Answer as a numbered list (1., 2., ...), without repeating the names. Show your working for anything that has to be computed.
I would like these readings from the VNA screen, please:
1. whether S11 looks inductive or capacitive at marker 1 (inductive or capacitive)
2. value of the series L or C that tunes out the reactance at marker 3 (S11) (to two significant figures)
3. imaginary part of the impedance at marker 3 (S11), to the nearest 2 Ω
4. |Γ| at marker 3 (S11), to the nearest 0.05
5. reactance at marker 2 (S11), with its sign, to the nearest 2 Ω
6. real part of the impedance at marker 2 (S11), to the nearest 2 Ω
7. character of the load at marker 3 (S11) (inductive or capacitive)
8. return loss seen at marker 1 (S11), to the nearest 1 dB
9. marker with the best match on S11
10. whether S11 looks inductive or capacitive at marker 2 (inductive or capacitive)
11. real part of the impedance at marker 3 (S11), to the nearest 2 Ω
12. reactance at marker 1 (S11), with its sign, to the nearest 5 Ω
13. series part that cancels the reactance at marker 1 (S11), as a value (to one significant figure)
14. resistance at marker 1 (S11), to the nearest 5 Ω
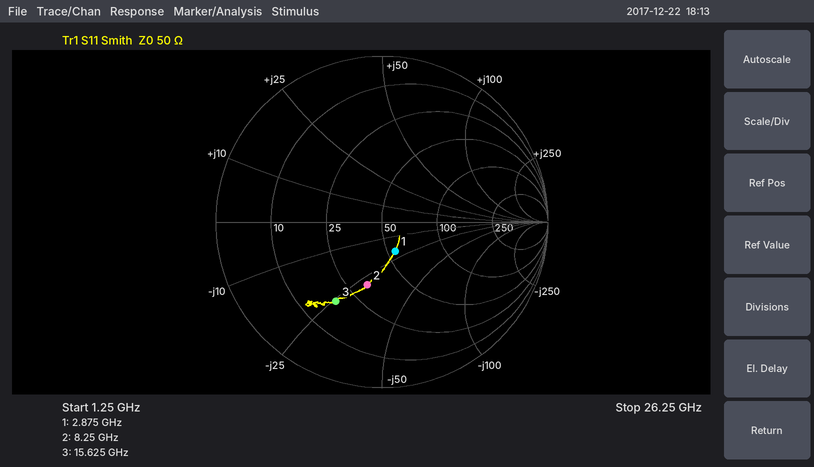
1. capacitive
2. L = 26 Ω/(2π × 15.625 GHz) ≈ 265 pH, so 260 pH to two significant figures
3. -26 Ω
4. 0.55
5. -28 Ω
6. 32 Ω
7. capacitive
8. 14 dB
9. marker 1
10. capacitive
11. 18 Ω
12. -20 Ω
13. L = 20 Ω/(2π × 2.875 GHz) ≈ 1 nH
14. 55 Ω
